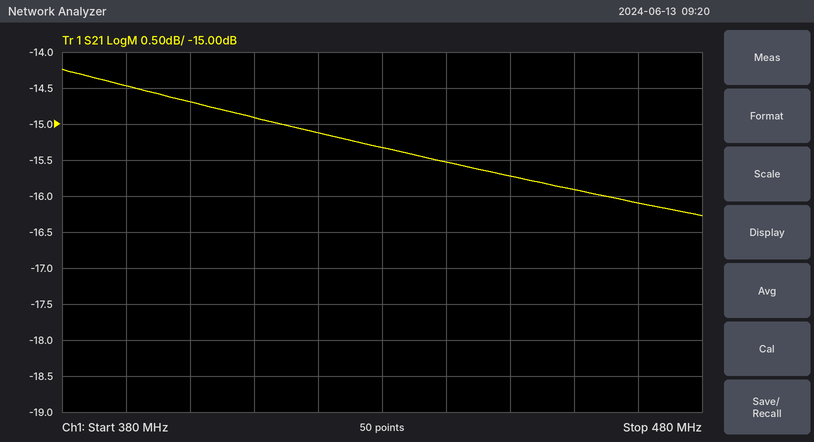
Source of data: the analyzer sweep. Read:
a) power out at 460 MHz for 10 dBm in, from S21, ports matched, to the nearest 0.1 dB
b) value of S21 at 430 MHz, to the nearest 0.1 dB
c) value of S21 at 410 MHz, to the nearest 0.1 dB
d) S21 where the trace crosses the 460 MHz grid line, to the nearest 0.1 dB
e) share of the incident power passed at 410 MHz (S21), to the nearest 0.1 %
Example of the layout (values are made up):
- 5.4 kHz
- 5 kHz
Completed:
- -5.9 dBm
- -15.3 dB
- -14.9 dB
- -15.9 dB
- 3.2 %
